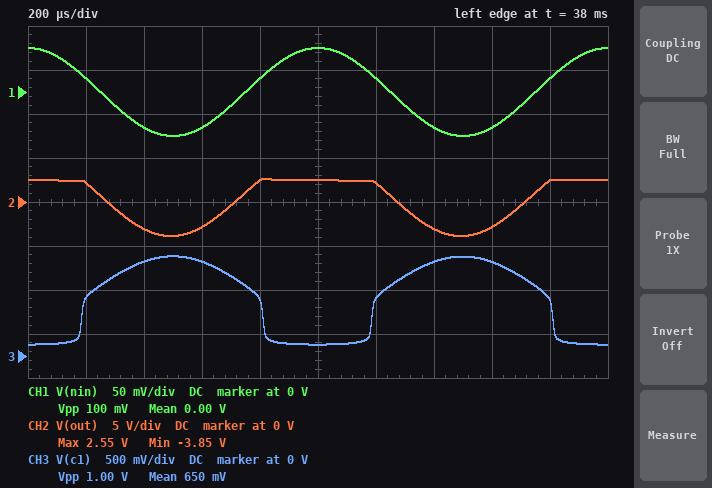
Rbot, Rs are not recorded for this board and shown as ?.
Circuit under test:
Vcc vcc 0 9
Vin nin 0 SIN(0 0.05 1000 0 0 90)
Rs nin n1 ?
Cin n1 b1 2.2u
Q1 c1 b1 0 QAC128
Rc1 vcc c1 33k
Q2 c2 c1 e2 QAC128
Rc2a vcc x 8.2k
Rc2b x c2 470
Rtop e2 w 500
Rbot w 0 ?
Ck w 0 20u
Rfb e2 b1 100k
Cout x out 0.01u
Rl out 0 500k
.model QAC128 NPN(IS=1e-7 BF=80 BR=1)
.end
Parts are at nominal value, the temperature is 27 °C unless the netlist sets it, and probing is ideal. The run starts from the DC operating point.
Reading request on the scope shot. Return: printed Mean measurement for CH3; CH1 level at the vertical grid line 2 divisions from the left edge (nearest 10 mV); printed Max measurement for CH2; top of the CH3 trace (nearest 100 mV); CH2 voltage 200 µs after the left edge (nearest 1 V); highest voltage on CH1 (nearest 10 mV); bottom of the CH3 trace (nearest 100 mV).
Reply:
650 mV
-40 mV
2.55 V
1.1 V
2 V
50 mV
100 mV
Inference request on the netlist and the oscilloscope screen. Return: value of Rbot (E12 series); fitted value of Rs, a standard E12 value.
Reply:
1.5 kΩ
15 kΩ
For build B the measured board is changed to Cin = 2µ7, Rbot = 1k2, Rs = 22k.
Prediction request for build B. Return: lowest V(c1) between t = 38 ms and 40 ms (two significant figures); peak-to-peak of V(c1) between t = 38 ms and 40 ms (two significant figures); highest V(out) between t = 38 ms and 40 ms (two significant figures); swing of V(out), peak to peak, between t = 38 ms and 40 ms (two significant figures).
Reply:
190 mV
860 mV
2.9 V
6.0 V
